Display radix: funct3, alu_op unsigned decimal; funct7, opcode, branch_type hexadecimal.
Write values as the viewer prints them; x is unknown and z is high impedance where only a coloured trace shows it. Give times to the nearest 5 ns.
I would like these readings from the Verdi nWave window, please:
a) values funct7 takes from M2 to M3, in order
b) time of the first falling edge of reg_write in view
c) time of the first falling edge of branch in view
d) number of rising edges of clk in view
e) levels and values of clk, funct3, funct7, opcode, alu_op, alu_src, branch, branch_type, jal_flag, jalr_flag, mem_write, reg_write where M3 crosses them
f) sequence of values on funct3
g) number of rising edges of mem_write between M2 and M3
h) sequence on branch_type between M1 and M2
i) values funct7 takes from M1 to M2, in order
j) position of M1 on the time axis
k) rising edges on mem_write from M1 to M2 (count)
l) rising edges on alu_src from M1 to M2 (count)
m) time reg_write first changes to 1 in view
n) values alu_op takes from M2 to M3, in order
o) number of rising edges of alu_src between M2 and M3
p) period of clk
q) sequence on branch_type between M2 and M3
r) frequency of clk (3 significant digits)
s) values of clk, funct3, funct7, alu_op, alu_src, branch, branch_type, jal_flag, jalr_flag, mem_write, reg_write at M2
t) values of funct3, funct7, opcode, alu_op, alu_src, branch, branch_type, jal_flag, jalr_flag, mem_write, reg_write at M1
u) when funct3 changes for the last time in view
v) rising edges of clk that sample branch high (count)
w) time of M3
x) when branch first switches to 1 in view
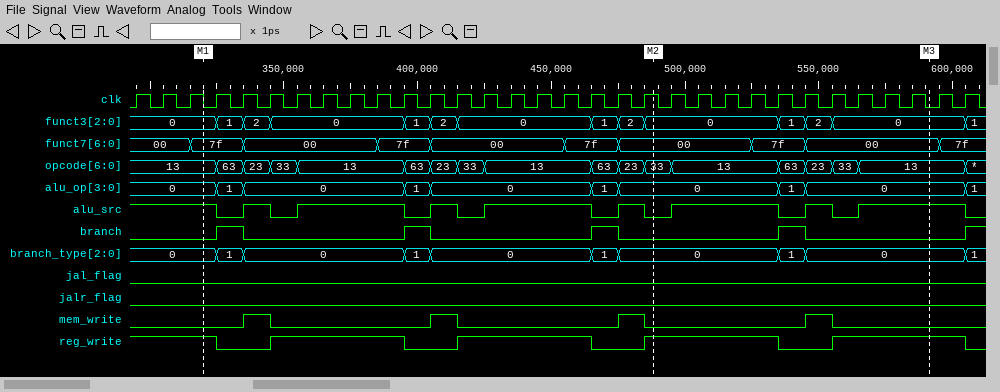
00, 7f, 00
325 ns
335 ns
32
clk=0, funct3=0, funct7=00, opcode=13, alu_op=0, alu_src=1, branch=0, branch_type=0, jal_flag=0, jalr_flag=0, mem_write=0, reg_write=1
0, 1, 2, 0, 1, 2, 0, 1, 2, 0, 1, 2, 0, 1
1
0, 1, 0, 1, 0, 1, 0
7f, 00, 7f, 00, 7f, 00
320 ns
3
5
345 ns
0, 1, 0
3
10 ns
0, 1, 0
100 MHz
clk=1, funct3=0, funct7=00, alu_op=0, alu_src=0, branch=0, branch_type=0, jal_flag=0, jalr_flag=0, mem_write=0, reg_write=1
funct3=0, funct7=7f, opcode=13, alu_op=0, alu_src=1, branch=0, branch_type=0, jal_flag=0, jalr_flag=0, mem_write=0, reg_write=1
605 ns
4
590 ns
325 ns
